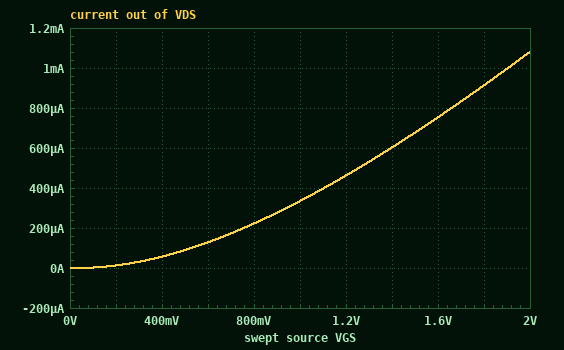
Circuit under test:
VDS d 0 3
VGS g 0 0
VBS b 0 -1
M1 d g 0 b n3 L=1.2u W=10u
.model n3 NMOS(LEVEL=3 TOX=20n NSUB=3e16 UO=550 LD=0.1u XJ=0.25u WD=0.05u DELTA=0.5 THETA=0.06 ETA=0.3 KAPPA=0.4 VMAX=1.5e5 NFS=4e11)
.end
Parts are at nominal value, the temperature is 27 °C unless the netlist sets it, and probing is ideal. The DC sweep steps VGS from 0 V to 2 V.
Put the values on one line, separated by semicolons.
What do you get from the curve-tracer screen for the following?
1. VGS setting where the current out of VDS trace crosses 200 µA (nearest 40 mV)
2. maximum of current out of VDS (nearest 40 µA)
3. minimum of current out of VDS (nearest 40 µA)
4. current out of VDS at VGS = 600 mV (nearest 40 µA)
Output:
760 mV; 1.08 mA; 0 A; 120 µA
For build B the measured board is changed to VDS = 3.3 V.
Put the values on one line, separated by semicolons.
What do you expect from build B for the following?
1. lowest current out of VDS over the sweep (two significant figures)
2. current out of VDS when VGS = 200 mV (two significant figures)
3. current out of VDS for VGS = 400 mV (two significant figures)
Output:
380 nA; 20 µA; 71 µA
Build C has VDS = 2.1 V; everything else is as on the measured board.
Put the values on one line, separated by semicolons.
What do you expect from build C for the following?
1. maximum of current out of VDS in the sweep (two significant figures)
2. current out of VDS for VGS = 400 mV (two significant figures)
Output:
930 µA; 25 µA
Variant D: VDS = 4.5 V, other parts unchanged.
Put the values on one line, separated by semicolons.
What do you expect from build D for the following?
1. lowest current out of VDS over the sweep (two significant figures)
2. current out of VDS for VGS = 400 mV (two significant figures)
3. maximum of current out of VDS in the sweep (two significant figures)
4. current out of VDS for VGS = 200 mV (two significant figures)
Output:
15 µA; 140 µA; 1.4 mA; 64 µA
